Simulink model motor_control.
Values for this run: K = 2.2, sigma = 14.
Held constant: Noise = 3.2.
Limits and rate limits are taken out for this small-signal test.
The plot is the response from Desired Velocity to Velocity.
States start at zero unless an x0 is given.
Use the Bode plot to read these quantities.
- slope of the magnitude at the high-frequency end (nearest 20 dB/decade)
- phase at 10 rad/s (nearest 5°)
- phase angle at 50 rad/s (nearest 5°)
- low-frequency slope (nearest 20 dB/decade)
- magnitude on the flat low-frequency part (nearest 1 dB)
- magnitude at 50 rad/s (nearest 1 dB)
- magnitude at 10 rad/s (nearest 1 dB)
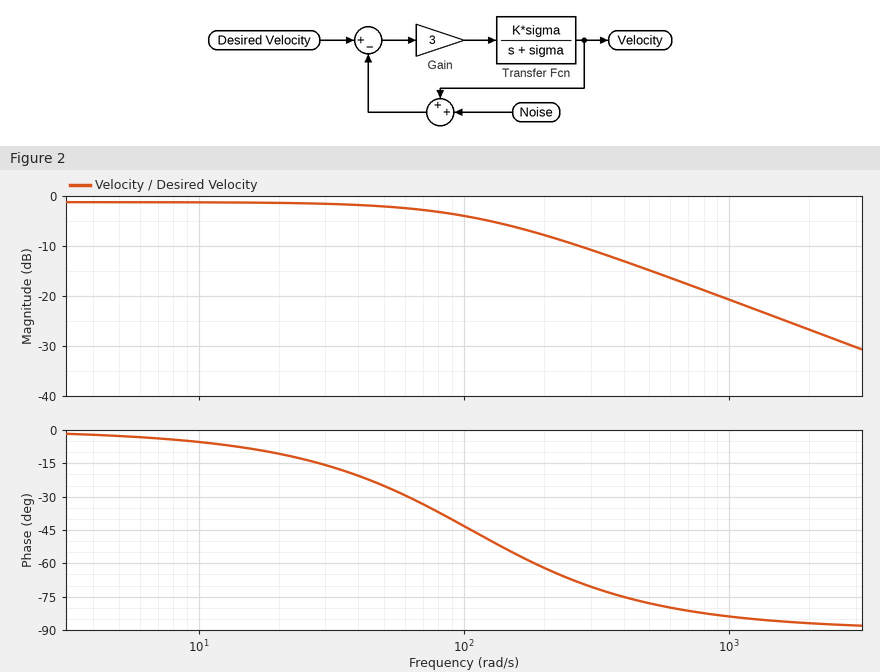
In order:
-20 dB/decade
-5°
-25°
0 dB/decade
-1 dB
-2 dB
-1 dB
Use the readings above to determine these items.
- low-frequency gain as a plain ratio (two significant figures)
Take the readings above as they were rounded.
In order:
0.89
